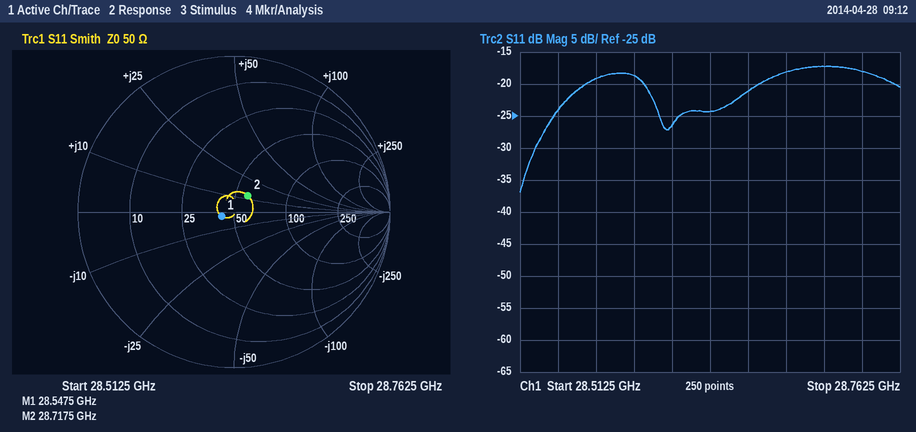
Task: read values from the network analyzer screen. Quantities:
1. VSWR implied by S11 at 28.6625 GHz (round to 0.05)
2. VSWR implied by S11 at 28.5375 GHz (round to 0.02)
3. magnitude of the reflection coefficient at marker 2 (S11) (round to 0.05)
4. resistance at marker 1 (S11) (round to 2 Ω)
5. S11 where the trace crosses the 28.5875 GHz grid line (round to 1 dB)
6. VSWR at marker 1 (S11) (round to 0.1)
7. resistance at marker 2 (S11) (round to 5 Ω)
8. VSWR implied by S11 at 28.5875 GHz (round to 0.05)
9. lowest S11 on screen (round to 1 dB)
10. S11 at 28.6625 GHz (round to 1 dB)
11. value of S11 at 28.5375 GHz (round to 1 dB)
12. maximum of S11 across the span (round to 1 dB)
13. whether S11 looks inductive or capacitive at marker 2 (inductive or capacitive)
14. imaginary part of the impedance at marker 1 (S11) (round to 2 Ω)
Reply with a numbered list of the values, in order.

1. 1.20
2. 1.14
3. 0.15
4. 42 Ω
5. -19 dB
6. 1.2
7. 60 Ω
8. 1.25
9. -37 dB
10. -21 dB
11. -24 dB
12. -17 dB
13. inductive
14. -2 Ω
